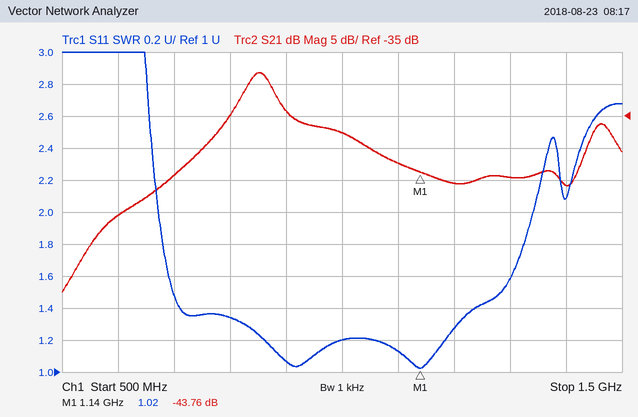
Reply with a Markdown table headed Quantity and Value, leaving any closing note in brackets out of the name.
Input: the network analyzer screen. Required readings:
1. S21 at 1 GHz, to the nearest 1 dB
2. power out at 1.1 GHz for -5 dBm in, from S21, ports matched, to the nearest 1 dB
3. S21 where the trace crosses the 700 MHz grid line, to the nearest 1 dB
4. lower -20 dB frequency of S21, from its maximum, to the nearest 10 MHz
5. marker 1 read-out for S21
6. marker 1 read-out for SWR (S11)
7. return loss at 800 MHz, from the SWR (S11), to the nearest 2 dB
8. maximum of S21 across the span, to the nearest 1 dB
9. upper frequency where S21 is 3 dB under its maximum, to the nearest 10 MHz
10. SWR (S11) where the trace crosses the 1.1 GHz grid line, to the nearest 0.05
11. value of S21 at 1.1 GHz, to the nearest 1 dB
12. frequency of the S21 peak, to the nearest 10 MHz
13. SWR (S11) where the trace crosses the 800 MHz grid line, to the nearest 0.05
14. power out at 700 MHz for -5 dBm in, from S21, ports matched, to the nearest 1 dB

| Quantity | Value |
|---|---|
| S21 at 1 GHz, to the nearest 1 dB | -38 dB |
| power out at 1.1 GHz for -5 dBm in, from S21, ports matched, to the nearest 1 dB | -47 dBm |
| S21 where the trace crosses the 700 MHz grid line, to the nearest 1 dB | -44 dB |
| lower -20 dB frequency of S21, from its maximum, to the nearest 10 MHz | 640 MHz |
| marker 1 read-out for S21 | -43.76 dB |
| marker 1 read-out for SWR | 1.02 |
| return loss at 800 MHz, from the SWR (S11), to the nearest 2 dB | 16 dB |
| maximum of S21 across the span, to the nearest 1 dB | -28 dB |
| upper frequency where S21 is 3 dB under its maximum, to the nearest 10 MHz | 880 MHz |
| SWR (S11) where the trace crosses the 1.1 GHz grid line, to the nearest 0.05 | 1.15 |
| value of S21 at 1.1 GHz, to the nearest 1 dB | -42 dB |
| frequency of the S21 peak, to the nearest 10 MHz | 850 MHz |
| SWR (S11) where the trace crosses the 800 MHz grid line, to the nearest 0.05 | 1.35 |
| power out at 700 MHz for -5 dBm in, from S21, ports matched, to the nearest 1 dB | -49 dBm |
